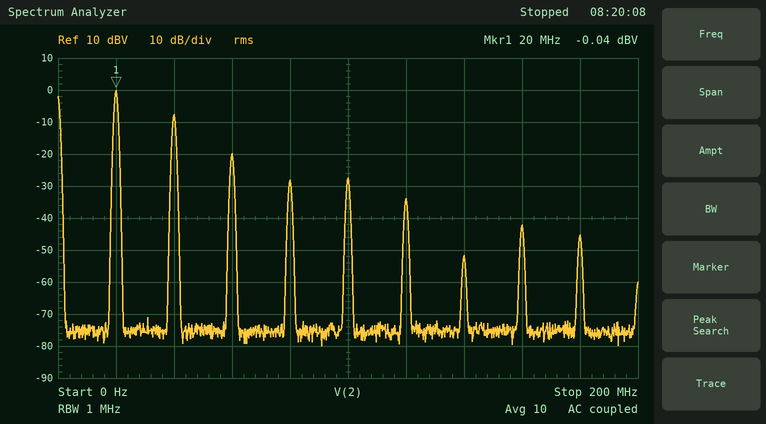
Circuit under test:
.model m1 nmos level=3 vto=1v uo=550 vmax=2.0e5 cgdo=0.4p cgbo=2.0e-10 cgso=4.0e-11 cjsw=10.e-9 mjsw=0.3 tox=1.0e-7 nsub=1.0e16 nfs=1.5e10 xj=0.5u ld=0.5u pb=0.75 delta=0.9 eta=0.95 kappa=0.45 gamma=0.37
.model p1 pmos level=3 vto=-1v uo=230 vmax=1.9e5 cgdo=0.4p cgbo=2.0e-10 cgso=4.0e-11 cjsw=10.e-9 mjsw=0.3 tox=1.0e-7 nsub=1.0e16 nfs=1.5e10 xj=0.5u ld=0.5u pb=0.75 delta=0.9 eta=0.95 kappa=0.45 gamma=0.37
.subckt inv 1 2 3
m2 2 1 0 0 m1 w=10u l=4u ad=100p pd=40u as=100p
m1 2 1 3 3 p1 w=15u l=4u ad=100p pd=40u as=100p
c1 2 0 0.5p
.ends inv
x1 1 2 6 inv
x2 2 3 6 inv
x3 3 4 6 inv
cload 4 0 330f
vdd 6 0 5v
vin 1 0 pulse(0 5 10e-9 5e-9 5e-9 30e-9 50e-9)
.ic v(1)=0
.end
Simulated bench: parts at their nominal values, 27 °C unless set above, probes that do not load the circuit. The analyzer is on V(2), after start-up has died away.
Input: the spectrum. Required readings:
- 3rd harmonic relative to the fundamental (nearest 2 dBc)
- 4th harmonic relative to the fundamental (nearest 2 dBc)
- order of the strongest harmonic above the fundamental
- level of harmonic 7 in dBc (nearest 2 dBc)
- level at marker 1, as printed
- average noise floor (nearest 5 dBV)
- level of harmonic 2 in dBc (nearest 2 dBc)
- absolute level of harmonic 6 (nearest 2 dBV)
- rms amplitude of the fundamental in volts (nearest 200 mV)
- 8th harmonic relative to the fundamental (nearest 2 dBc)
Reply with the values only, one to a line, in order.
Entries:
-20 dBc
-28 dBc
2
-52 dBc
-0.04 dBV
-75 dBV
-8 dBc
-34 dBV
1.0 V
-42 dBc
